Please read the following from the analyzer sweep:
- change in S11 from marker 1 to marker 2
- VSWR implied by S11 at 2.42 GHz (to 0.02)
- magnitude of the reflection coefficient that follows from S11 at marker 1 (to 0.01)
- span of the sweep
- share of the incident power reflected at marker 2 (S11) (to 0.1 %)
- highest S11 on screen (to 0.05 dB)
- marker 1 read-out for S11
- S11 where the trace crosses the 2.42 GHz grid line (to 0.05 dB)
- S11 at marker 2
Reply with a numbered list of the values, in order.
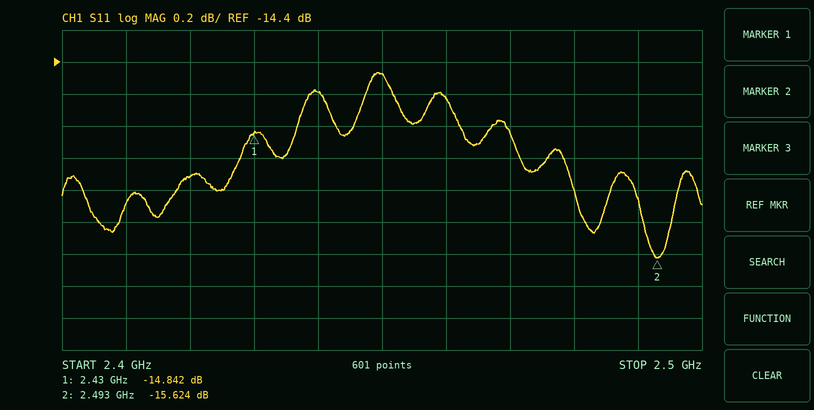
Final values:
1. -0.782 dB
2. 1.42
3. 0.18
4. 100 MHz
5. 2.7 %
6. -14.45 dB
7. -14.842 dB
8. -15.10 dB
9. -15.624 dB
